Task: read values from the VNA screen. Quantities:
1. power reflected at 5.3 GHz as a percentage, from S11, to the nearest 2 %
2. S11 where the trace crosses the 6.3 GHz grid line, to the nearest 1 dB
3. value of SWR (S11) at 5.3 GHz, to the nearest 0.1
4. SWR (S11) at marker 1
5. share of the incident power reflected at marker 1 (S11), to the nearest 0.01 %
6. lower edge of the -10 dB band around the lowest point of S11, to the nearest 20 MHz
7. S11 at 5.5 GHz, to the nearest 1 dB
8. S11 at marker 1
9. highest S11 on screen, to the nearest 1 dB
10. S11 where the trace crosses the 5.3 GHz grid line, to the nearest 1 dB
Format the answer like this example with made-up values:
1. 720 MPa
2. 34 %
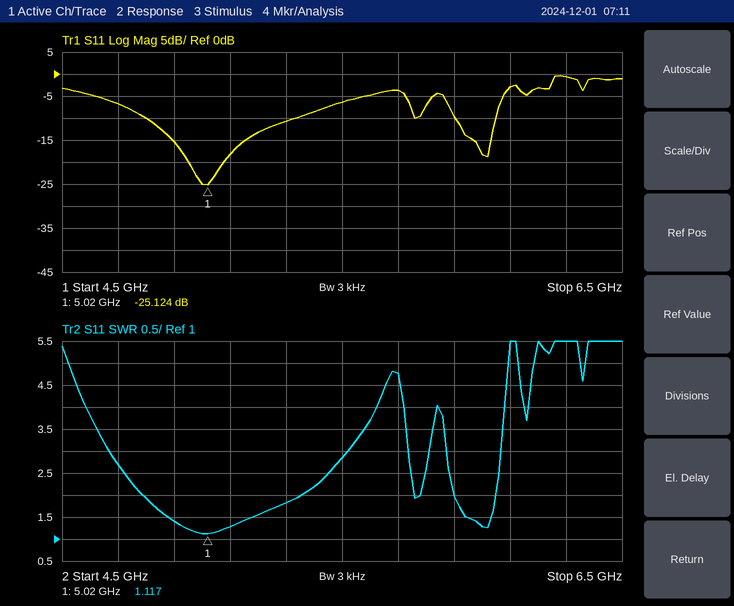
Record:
1. 8 %
2. -1 dB
3. 1.8
4. 1.117
5. 0.31 %
6. 4.80 GHz
7. -6 dB
8. -25.124 dB
9. 0 dB
10. -11 dB
